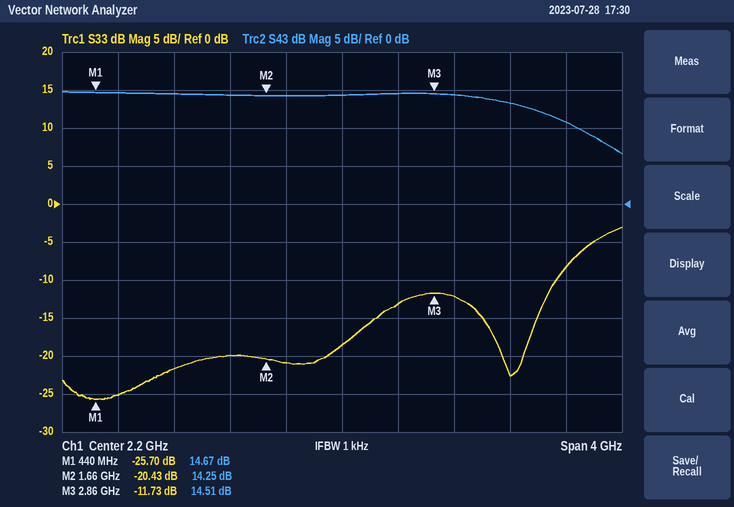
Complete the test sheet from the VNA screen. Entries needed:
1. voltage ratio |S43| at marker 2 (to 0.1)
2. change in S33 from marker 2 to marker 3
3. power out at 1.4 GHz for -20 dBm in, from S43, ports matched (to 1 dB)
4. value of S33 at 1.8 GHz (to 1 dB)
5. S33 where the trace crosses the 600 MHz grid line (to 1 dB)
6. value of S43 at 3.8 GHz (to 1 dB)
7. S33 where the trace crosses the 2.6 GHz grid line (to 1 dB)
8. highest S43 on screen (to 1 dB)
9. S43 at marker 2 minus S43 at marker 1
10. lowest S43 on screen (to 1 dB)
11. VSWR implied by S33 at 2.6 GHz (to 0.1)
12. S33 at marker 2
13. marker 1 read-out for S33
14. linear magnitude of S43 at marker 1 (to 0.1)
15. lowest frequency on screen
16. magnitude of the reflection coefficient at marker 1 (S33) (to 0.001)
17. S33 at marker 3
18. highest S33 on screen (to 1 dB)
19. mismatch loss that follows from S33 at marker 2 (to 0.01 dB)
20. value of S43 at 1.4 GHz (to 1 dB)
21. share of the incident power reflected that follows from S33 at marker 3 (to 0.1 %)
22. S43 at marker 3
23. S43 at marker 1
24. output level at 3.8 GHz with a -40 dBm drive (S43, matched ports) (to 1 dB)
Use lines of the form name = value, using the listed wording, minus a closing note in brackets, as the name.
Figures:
voltage ratio |S43| at marker 2 = 5.2
change in S33 from marker 2 to marker 3 = 8.70 dB
power out at 1.4 GHz for -20 dBm in, from S43, ports matched = -6 dBm
value of S33 at 1.8 GHz = -21 dB
S33 where the trace crosses the 600 MHz grid line = -25 dB
value of S43 at 3.8 GHz = 11 dB
S33 where the trace crosses the 2.6 GHz grid line = -13 dB
highest S43 on screen = 15 dB
S43 at marker 2 minus S43 at marker 1 = -0.42 dB
lowest S43 on screen = 7 dB
VSWR implied by S33 at 2.6 GHz = 1.6
S33 at marker 2 = -20.43 dB
marker 1 read-out for S33 = -25.70 dB
linear magnitude of S43 at marker 1 = 5.4
lowest frequency on screen = 200 MHz
magnitude of the reflection coefficient at marker 1 (S33) = 0.052
S33 at marker 3 = -11.73 dB
highest S33 on screen = -3 dB
mismatch loss that follows from S33 at marker 2 = 0.04 dB
value of S43 at 1.4 GHz = 14 dB
share of the incident power reflected that follows from S33 at marker 3 = 6.7 %
S43 at marker 3 = 14.51 dB
S43 at marker 1 = 14.67 dB
output level at 3.8 GHz with a -40 dBm drive (S43, matched ports) = -29 dBm
